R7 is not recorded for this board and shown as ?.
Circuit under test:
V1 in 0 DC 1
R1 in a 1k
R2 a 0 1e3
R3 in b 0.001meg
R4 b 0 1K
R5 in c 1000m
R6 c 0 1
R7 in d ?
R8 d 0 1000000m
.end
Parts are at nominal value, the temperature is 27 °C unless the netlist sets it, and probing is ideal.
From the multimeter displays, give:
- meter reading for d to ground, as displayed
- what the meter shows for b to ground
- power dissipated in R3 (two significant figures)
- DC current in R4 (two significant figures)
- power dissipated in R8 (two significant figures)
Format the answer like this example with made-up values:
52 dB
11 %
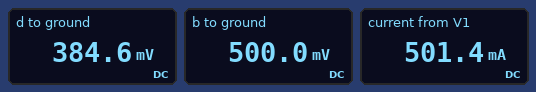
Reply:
384.6 mV
500.0 mV
250 µW
500 µA
150 µW
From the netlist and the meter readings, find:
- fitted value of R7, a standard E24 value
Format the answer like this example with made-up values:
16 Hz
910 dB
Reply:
1.6 kΩ
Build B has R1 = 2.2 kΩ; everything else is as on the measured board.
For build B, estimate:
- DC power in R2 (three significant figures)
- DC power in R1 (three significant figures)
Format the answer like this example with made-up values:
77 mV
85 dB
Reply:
97.7 µW
215 µW
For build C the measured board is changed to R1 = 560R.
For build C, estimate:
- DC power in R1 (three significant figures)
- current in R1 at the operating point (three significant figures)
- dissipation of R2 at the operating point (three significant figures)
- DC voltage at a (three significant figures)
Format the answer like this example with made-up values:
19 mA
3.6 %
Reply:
230 µW
641 µA
411 µW
641 mV
